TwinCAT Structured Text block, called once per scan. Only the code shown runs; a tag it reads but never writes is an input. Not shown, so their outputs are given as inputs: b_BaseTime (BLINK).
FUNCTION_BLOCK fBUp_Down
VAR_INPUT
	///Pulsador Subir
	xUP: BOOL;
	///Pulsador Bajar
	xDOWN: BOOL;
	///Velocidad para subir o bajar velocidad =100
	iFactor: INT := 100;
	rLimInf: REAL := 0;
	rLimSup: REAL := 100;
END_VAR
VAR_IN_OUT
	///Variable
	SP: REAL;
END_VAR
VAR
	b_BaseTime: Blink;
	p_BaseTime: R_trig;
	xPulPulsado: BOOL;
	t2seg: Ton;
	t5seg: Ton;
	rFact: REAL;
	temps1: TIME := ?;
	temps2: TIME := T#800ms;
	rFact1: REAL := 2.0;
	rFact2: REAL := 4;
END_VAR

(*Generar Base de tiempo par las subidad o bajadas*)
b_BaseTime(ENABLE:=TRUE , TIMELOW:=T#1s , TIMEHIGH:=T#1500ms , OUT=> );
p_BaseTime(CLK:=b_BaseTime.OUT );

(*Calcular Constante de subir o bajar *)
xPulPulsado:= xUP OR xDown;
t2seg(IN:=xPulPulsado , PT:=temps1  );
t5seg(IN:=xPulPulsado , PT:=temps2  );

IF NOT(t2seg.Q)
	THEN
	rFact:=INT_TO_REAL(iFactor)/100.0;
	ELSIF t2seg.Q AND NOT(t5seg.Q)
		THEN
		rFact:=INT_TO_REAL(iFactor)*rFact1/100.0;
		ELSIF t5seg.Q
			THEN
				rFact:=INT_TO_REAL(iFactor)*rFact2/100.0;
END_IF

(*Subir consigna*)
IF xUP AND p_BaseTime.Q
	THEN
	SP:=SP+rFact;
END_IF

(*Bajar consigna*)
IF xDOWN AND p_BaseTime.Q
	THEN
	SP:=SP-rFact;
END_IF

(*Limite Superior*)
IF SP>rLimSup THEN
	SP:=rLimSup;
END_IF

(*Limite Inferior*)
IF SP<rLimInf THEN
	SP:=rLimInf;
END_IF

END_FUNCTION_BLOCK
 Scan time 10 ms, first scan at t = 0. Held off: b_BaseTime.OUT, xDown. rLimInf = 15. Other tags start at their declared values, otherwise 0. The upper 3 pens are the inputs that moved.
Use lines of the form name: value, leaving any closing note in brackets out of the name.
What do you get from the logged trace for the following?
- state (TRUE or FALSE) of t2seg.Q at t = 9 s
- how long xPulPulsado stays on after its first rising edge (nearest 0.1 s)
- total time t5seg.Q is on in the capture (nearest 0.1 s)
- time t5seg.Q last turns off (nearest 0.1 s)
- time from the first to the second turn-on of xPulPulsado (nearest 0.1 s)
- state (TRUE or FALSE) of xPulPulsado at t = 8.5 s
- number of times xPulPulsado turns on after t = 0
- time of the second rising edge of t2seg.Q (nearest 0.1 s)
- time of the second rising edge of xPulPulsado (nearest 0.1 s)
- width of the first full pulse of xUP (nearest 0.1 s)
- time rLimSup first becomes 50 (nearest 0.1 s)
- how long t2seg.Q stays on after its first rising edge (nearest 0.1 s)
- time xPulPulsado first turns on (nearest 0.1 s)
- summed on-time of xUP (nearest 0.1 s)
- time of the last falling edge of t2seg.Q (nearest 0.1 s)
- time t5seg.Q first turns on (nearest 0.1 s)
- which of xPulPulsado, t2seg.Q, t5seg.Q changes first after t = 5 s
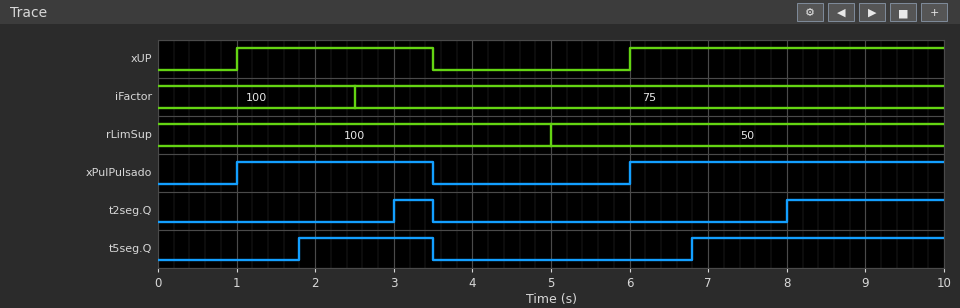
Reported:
state (TRUE or FALSE) of t2seg.Q at t = 9 s: TRUE
how long xPulPulsado stays on after its first rising edge: 2.5 s
total time t5seg.Q is on in the capture: 4.9 s
time t5seg.Q last turns off: 3.5 s
time from the first to the second turn-on of xPulPulsado: 5.0 s
state (TRUE or FALSE) of xPulPulsado at t = 8.5 s: TRUE
number of times xPulPulsado turns on after t = 0: 2
time of the second rising edge of t2seg.Q: 8.0 s
time of the second rising edge of xPulPulsado: 6.0 s
width of the first full pulse of xUP: 2.5 s
time rLimSup first becomes 50: 5.0 s
how long t2seg.Q stays on after its first rising edge: 0.5 s
time xPulPulsado first turns on: 1.0 s
summed on-time of xUP: 6.5 s
time of the last falling edge of t2seg.Q: 3.5 s
time t5seg.Q first turns on: 1.8 s
which of xPulPulsado, t2seg.Q, t5seg.Q changes first after t = 5 s: xPulPulsado
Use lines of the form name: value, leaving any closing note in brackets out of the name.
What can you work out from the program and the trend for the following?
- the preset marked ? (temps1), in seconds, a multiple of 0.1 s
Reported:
the preset marked ? (temps1), in seconds, a multiple of 0.1 s: 2.0 s
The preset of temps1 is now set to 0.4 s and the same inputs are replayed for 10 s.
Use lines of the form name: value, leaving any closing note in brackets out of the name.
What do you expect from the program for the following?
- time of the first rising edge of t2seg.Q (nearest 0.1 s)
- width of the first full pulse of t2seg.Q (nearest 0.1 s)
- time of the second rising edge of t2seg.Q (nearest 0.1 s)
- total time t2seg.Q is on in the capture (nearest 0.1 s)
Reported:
time of the first rising edge of t2seg.Q: 1.4 s
width of the first full pulse of t2seg.Q: 2.1 s
time of the second rising edge of t2seg.Q: 6.4 s
total time t2seg.Q is on in the capture: 5.7 s
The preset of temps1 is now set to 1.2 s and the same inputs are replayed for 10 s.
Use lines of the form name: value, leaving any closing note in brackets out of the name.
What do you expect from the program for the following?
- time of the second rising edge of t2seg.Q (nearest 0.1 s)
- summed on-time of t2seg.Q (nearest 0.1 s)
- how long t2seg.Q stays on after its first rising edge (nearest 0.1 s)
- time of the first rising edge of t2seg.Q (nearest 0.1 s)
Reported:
time of the second rising edge of t2seg.Q: 7.2 s
summed on-time of t2seg.Q: 4.1 s
how long t2seg.Q stays on after its first rising edge: 1.3 s
time of the first rising edge of t2seg.Q: 2.2 s
